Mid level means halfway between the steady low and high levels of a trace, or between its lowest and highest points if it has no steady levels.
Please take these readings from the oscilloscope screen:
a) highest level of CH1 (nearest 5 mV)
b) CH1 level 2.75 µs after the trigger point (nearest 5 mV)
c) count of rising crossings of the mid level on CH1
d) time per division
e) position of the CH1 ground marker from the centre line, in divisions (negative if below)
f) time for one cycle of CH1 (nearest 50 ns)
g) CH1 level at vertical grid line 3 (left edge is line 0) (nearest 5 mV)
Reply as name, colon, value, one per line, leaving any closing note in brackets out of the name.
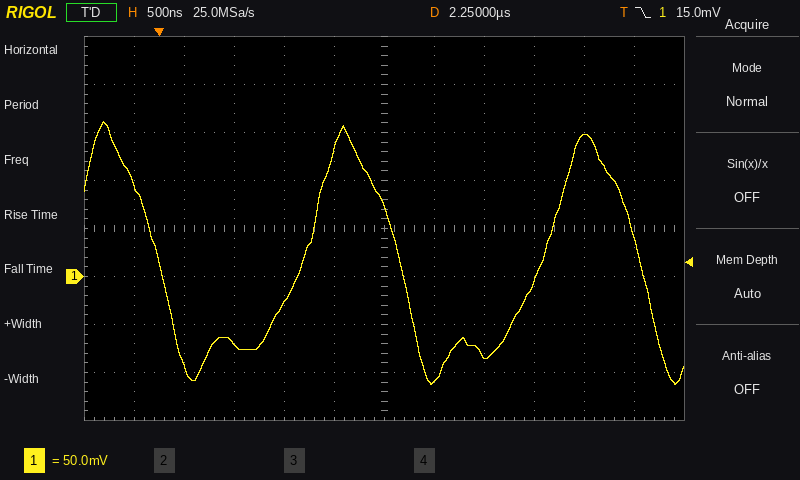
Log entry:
highest level of CH1: 160 mV
CH1 level 2.75 µs after the trigger point: -110 mV
count of rising crossings of the mid level on CH1: 2
time per division: 500 ns
position of the CH1 ground marker from the centre line, in divisions: -1.0 div
time for one cycle of CH1: 2.40 µs
CH1 level at vertical grid line 3 (left edge is line 0): -70 mV
